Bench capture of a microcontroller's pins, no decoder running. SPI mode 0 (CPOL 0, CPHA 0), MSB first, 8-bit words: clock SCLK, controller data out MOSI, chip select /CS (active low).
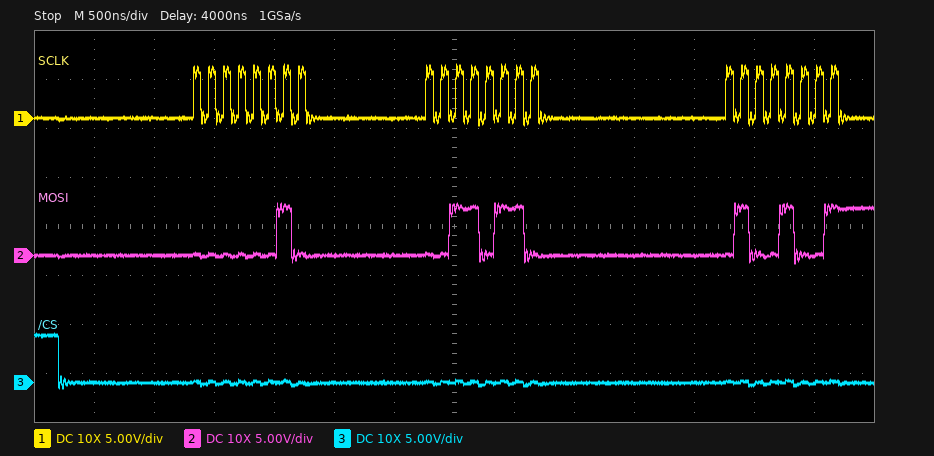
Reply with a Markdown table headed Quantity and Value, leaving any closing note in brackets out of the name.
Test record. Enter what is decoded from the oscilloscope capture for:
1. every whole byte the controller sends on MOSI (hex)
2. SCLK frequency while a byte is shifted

| Quantity | Value |
|---|---|
| every whole byte the controller sends on MOSI | 0x02 0x36 0x49 |
| SCLK frequency while a byte is shifted | 8 MHz |
